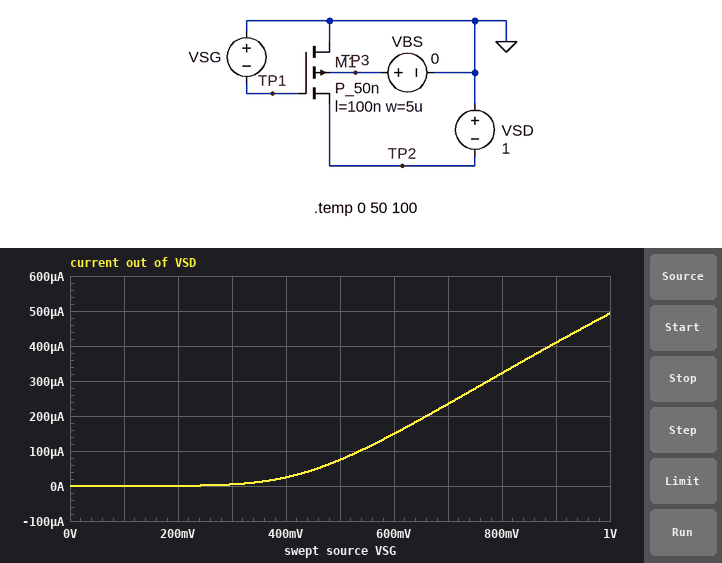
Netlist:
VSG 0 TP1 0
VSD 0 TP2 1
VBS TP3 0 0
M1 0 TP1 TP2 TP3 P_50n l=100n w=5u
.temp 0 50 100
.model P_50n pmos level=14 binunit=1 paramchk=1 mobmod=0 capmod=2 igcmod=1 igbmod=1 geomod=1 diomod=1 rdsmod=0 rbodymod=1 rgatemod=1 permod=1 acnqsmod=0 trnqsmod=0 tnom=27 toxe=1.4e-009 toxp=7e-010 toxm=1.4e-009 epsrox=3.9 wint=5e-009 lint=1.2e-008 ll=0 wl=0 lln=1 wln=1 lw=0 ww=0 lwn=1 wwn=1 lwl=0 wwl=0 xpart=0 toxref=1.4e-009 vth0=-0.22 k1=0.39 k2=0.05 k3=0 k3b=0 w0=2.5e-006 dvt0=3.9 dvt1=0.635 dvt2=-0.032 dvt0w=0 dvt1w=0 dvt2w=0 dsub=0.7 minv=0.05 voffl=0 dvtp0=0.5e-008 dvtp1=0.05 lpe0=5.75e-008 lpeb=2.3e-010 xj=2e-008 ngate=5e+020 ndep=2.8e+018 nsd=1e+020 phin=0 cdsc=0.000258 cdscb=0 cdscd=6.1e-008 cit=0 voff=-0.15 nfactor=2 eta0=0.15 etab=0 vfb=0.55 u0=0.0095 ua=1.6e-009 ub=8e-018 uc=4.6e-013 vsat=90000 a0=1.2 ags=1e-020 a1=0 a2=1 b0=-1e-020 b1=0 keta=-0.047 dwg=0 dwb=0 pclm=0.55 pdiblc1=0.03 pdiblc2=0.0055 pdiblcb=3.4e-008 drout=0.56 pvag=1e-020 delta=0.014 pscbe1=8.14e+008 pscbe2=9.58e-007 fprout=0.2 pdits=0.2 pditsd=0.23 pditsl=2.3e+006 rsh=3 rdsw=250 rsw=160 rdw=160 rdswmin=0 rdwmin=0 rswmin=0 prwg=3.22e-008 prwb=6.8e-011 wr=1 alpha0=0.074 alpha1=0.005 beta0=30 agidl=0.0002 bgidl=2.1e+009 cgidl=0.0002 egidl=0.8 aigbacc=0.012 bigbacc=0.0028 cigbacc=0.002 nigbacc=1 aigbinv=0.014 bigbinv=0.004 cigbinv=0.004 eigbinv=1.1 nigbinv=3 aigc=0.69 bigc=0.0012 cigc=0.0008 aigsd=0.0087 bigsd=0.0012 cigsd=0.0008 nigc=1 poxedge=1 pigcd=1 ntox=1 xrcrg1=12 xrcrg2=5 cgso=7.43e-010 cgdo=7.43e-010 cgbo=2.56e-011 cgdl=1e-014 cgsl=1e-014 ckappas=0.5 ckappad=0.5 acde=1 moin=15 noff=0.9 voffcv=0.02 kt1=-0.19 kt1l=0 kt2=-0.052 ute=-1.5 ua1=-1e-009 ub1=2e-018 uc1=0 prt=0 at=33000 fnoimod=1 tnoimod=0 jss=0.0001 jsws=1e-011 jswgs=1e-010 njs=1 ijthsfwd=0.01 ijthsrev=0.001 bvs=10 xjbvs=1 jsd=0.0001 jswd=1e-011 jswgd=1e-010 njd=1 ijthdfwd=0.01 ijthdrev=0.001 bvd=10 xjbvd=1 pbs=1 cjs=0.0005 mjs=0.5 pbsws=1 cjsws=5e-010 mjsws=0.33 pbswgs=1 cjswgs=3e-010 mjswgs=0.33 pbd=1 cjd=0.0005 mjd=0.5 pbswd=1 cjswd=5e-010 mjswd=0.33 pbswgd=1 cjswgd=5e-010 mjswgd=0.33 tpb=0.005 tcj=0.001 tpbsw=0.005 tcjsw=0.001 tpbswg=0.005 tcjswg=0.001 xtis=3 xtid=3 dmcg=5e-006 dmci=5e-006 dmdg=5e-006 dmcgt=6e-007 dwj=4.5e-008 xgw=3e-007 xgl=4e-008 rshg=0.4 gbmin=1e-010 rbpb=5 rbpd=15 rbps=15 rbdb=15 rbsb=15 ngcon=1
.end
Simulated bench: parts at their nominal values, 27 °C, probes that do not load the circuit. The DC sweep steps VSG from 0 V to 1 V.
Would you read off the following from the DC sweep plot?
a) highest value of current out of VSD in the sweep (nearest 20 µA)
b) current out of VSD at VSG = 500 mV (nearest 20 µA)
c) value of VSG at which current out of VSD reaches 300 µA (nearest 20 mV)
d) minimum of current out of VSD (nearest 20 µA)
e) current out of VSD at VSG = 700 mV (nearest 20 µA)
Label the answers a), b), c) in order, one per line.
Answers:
a) 500 µA
b) 80 µA
c) 780 mV
d) 0 A
e) 240 µA
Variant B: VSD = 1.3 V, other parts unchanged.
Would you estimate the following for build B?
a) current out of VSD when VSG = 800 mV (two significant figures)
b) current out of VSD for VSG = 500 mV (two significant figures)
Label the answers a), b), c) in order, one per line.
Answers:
a) 340 µA
b) 80 µA
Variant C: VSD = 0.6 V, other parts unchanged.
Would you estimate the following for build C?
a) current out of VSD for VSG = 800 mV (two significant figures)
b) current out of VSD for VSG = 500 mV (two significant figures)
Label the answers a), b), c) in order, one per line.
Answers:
a) 300 µA
b) 69 µA
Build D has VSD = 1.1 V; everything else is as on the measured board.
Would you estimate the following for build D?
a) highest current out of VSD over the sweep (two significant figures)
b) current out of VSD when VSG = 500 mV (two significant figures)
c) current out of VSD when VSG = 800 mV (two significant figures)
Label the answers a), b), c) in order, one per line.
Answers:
a) 500 µA
b) 76 µA
c) 330 µA
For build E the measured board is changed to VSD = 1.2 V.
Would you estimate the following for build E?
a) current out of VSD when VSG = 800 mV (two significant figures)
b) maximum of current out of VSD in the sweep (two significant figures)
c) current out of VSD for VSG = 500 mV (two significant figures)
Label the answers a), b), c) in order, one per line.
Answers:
a) 330 µA
b) 510 µA
c) 78 µA
